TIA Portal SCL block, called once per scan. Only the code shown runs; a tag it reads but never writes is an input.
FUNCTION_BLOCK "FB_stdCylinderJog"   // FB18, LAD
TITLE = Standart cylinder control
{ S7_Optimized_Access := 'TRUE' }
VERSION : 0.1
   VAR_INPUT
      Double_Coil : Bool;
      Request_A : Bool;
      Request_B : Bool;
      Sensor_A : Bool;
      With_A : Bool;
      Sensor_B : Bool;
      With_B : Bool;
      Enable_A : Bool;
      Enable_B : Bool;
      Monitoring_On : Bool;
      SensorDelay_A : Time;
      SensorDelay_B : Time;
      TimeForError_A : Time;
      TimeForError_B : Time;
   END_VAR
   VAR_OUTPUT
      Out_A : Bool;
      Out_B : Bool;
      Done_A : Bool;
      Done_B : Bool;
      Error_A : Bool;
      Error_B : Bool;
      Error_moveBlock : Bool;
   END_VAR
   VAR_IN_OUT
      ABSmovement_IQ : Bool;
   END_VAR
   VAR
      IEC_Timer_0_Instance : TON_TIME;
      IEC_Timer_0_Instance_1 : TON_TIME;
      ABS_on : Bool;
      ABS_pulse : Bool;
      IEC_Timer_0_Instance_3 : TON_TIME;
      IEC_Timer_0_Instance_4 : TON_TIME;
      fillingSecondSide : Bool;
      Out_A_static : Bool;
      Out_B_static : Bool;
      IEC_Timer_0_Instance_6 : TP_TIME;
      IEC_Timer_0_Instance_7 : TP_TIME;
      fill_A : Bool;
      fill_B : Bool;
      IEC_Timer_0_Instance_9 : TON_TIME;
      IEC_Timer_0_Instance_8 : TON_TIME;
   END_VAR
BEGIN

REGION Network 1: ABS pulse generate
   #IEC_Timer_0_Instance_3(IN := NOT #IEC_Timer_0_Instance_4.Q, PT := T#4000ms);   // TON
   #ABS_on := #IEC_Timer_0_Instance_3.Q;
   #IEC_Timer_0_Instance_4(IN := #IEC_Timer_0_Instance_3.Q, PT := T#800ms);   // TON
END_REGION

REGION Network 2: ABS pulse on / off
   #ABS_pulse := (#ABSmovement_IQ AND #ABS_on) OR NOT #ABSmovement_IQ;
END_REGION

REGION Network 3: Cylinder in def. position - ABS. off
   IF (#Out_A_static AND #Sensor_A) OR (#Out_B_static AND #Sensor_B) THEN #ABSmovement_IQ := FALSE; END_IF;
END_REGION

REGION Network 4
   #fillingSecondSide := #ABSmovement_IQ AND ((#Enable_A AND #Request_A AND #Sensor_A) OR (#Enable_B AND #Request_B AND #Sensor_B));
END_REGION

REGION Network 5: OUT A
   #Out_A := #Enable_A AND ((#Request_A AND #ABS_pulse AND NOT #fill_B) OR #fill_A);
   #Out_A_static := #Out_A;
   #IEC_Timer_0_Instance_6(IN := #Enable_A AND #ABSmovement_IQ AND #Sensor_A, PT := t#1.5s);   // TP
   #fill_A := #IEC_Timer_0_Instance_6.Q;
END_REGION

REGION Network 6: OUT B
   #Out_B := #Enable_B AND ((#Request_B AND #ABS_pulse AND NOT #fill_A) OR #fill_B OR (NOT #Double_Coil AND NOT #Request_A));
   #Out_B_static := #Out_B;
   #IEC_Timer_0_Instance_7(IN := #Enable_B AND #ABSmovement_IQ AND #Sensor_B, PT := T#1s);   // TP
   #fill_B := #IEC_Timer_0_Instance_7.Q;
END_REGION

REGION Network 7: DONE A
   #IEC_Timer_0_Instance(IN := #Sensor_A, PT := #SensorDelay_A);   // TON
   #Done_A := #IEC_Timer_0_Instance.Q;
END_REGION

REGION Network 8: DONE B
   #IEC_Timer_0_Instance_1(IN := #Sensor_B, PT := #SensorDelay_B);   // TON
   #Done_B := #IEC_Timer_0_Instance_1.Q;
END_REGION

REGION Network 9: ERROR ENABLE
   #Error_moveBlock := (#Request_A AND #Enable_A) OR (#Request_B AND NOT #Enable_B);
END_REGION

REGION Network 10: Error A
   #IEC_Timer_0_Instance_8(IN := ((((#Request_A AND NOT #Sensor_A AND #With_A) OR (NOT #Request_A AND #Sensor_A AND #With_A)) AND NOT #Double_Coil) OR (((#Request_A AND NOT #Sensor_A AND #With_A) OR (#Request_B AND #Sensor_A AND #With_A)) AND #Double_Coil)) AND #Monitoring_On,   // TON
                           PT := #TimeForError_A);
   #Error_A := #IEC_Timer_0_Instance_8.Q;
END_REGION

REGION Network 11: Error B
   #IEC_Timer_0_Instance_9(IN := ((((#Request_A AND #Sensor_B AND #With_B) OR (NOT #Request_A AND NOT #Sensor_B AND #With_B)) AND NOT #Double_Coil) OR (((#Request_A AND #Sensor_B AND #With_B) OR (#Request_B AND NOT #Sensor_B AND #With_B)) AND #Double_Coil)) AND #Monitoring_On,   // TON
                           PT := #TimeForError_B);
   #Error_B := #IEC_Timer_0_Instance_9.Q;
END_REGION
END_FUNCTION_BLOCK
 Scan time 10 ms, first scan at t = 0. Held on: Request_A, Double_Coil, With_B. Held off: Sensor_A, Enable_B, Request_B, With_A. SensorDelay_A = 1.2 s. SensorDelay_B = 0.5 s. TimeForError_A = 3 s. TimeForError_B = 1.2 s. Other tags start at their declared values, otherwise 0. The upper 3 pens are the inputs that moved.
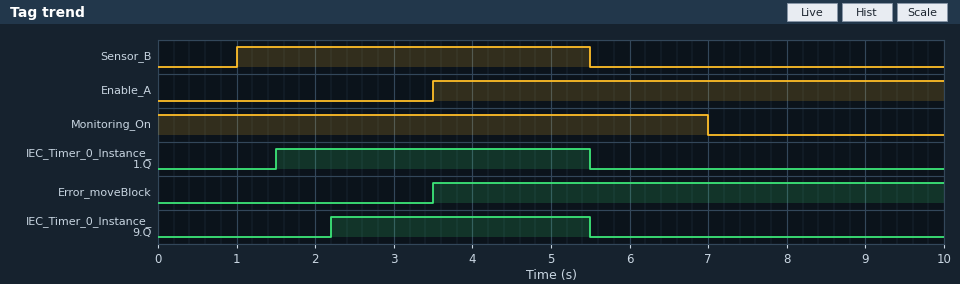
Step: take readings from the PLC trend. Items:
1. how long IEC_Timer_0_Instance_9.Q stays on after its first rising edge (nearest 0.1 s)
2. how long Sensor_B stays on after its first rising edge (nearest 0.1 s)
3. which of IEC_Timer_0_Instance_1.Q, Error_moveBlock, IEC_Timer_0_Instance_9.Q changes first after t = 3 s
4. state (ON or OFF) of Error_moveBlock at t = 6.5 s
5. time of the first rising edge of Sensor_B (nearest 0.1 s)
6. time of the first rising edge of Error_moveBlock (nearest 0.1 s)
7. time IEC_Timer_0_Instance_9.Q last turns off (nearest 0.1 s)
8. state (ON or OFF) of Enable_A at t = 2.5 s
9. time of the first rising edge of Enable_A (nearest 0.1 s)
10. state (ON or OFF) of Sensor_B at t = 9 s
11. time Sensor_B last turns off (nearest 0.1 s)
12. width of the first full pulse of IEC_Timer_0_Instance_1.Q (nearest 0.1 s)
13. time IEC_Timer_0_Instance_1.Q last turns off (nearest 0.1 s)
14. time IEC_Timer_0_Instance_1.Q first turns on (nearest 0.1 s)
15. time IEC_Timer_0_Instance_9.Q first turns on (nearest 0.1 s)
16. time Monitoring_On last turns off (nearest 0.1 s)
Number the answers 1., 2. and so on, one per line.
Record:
1. 3.3 s
2. 4.5 s
3. Error_moveBlock
4. ON
5. 1.0 s
6. 3.5 s
7. 5.5 s
8. OFF
9. 3.5 s
10. OFF
11. 5.5 s
12. 4.0 s
13. 5.5 s
14. 1.5 s
15. 2.2 s
16. 7.0 s
